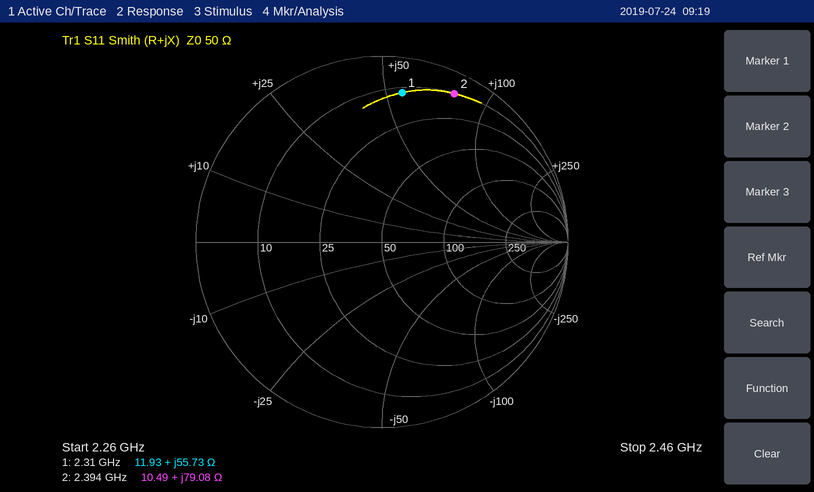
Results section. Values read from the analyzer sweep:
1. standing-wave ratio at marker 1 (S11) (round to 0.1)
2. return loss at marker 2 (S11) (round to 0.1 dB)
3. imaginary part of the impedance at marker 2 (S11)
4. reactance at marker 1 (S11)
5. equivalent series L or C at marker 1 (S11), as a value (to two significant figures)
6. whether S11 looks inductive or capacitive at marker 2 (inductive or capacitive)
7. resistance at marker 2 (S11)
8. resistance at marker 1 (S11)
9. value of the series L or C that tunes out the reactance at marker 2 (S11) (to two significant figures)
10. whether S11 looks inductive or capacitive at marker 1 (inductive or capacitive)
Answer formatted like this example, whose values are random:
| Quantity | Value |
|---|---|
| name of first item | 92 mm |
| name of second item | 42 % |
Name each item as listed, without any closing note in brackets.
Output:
| Quantity | Value |
|---|---|
| standing-wave ratio at marker 1 (S11) | 9.5 |
| return loss at marker 2 (S11) | 1.0 dB |
| imaginary part of the impedance at marker 2 | +79.08 Ω |
| reactance at marker 1 | +55.73 Ω |
| equivalent series L or C at marker 1 (S11), as a value | 3.8 nH |
| whether S11 looks inductive or capacitive at marker 2 | inductive |
| resistance at marker 2 | 10.49 Ω |
| resistance at marker 1 | 11.93 Ω |
| value of the series L or C that tunes out the reactance at marker 2 (S11) | 840 fF |
| whether S11 looks inductive or capacitive at marker 1 | inductive |
